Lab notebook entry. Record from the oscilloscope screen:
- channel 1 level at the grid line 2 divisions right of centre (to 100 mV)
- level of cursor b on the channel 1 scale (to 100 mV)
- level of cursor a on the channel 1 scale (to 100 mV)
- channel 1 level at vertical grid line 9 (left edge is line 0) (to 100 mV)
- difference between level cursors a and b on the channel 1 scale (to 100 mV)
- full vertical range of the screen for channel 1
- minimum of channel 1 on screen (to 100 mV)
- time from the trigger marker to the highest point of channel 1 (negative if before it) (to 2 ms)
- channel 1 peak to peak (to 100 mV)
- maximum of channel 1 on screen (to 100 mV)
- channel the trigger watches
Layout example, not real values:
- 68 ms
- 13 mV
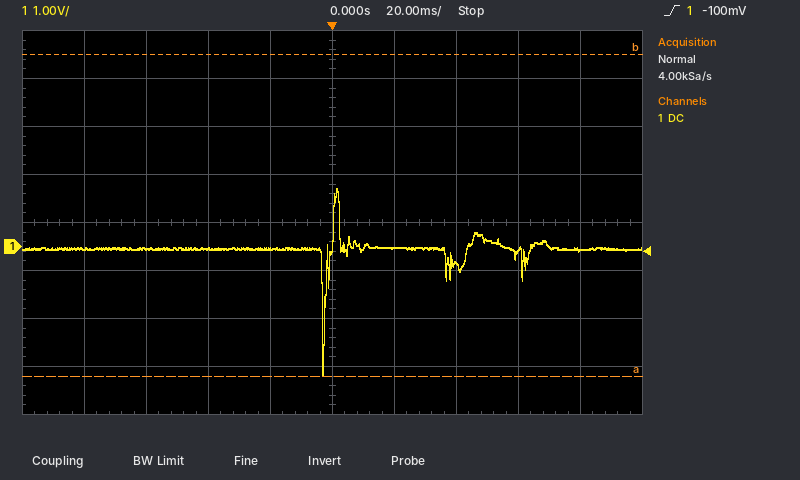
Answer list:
- -400 mV
- 4.0 V
- -2.7 V
- -100 mV
- 6.7 V
- 8 V
- -2.7 V
- +2 ms
- 3.9 V
- 1.2 V
- channel 1
